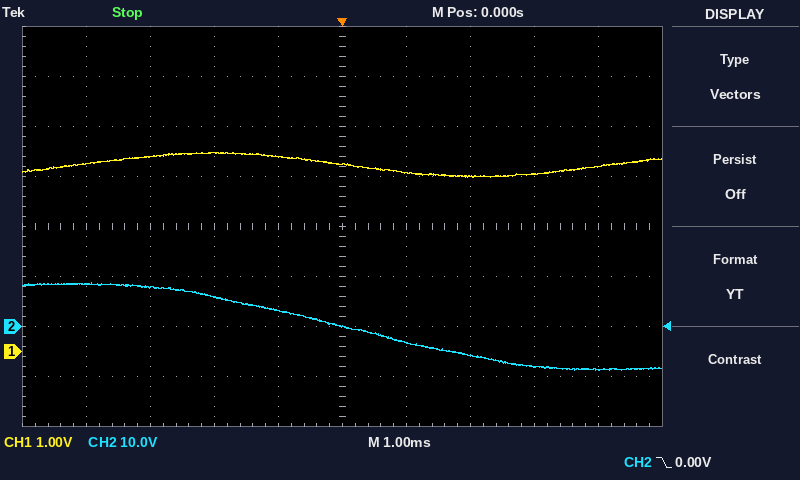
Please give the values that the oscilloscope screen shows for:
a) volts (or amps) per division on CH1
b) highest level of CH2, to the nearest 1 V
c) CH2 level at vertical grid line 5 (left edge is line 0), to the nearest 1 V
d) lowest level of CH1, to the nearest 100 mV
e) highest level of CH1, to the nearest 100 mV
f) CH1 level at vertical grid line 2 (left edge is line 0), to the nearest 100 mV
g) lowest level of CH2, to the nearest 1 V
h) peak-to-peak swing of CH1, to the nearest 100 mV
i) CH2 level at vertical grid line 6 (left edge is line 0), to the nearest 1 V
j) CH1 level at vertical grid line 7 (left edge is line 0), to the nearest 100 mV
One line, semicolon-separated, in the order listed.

1 V; 9 V; 0 V; 3.5 V; 4.0 V; 3.9 V; -9 V; 500 mV; -3 V; 3.5 V
